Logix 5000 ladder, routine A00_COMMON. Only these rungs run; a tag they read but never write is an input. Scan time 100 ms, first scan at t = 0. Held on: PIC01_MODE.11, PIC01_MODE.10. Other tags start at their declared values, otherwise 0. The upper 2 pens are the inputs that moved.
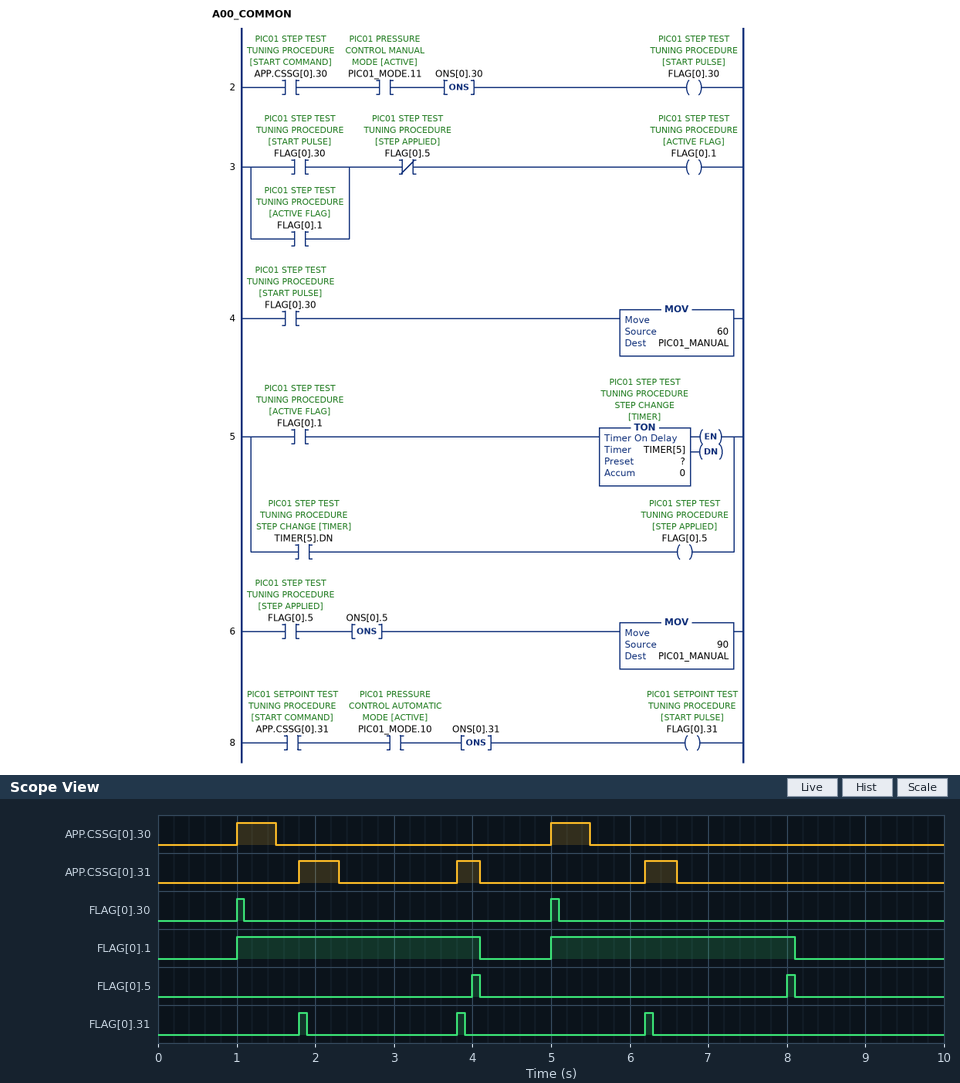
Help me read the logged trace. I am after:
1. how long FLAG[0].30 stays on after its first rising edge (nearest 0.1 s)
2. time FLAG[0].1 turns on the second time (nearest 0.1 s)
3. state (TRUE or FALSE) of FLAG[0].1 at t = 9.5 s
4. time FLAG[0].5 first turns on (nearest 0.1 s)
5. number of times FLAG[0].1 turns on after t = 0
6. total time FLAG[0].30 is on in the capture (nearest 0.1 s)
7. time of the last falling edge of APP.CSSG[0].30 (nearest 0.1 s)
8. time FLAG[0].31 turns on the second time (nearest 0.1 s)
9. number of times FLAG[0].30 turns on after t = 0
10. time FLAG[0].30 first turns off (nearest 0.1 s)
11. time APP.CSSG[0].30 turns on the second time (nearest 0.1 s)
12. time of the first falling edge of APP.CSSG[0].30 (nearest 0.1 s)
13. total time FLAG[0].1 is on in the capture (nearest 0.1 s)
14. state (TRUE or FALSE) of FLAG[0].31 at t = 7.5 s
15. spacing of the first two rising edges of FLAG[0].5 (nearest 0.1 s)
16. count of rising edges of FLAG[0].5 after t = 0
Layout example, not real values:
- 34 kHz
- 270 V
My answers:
- 0.1 s
- 5.0 s
- FALSE
- 4.0 s
- 2
- 0.2 s
- 5.5 s
- 3.8 s
- 2
- 1.1 s
- 5.0 s
- 1.5 s
- 6.2 s
- FALSE
- 4.0 s
- 2
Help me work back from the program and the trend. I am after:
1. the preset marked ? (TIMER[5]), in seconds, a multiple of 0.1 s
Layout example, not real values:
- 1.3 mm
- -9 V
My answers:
- 3.0 s
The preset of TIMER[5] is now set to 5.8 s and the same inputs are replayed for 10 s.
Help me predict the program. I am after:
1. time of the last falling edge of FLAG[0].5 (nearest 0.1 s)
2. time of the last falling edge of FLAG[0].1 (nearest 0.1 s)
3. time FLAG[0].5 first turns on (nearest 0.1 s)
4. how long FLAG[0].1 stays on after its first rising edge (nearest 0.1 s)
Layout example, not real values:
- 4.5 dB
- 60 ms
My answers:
- 6.9 s
- 6.9 s
- 6.8 s
- 5.9 s
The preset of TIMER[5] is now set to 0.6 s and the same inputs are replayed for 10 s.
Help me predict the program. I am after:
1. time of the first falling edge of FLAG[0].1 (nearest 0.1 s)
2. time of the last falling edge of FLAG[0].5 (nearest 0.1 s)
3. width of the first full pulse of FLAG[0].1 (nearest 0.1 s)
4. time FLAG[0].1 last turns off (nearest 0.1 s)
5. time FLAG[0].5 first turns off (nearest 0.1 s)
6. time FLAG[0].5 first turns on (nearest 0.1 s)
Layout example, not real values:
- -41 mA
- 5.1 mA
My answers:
- 1.7 s
- 5.7 s
- 0.7 s
- 5.7 s
- 1.7 s
- 1.6 s
